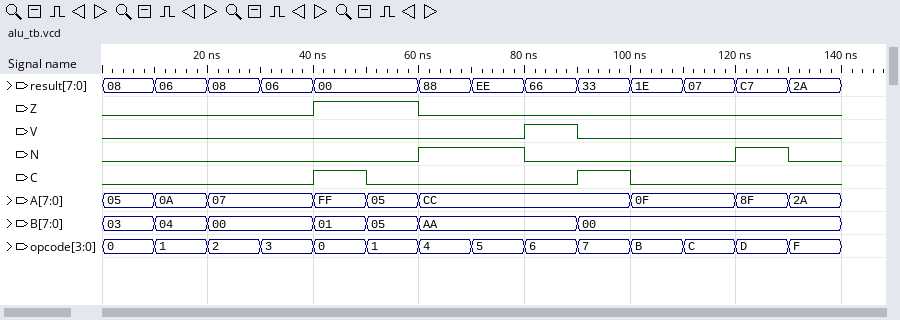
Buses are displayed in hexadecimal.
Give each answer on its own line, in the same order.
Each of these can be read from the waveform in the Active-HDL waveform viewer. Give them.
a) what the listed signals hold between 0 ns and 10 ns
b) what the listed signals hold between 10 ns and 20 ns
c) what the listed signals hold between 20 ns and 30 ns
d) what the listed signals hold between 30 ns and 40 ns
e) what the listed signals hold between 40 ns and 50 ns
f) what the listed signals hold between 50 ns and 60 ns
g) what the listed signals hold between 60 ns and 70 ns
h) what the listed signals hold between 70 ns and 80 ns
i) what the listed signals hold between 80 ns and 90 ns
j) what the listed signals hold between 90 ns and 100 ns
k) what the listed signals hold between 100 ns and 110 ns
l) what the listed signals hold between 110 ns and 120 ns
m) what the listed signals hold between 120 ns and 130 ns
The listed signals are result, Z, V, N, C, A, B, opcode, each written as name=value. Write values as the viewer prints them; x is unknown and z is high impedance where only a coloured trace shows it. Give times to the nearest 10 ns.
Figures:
result=08, Z=0, V=0, N=0, C=0, A=05, B=03, opcode=0
result=06, Z=0, V=0, N=0, C=0, A=0A, B=04, opcode=1
result=08, Z=0, V=0, N=0, C=0, A=07, B=00, opcode=2
result=06, Z=0, V=0, N=0, C=0, A=07, B=00, opcode=3
result=00, Z=1, V=0, N=0, C=1, A=FF, B=01, opcode=0
result=00, Z=1, V=0, N=0, C=0, A=05, B=05, opcode=1
result=88, Z=0, V=0, N=1, C=0, A=CC, B=AA, opcode=4
result=EE, Z=0, V=0, N=1, C=0, A=CC, B=AA, opcode=5
result=66, Z=0, V=1, N=0, C=0, A=CC, B=AA, opcode=6
result=33, Z=0, V=0, N=0, C=1, A=CC, B=00, opcode=7
result=1E, Z=0, V=0, N=0, C=0, A=0F, B=00, opcode=B
result=07, Z=0, V=0, N=0, C=0, A=0F, B=00, opcode=C
result=C7, Z=0, V=0, N=1, C=0, A=8F, B=00, opcode=D
